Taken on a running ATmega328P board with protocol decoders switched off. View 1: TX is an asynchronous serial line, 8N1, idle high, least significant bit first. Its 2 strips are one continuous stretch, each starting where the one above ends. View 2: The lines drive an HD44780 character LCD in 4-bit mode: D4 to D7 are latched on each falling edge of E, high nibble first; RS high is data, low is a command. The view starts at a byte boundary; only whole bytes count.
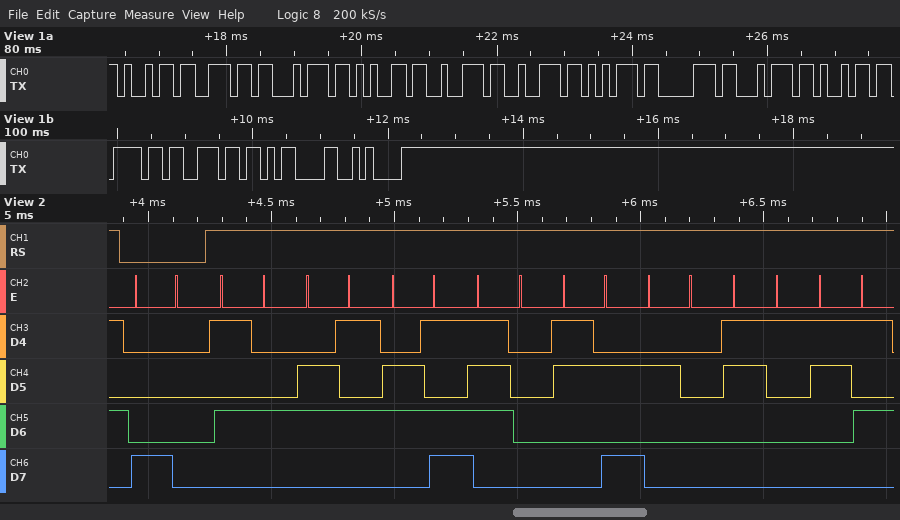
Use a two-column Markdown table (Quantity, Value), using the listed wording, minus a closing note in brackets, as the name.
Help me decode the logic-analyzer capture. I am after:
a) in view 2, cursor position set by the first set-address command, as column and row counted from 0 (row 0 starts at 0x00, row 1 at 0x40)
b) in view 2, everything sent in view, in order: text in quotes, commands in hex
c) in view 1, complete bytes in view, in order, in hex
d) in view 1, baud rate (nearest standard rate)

| Quantity | Value |
|---|---|
| in view 2, cursor position set by the first set-address command, as column and row counted from 0 | column 0, row 0 |
| in view 2, everything sent in view, in order: text in quotes, commands in hex | 0x80 "Temp: 15" |
| in view 1, complete bytes in view, in order, in hex | 69 6E 74 65 72 72 75 70 74 69 6F 6E 0D 0A |
| in view 1, baud rate | 9600 baud |
